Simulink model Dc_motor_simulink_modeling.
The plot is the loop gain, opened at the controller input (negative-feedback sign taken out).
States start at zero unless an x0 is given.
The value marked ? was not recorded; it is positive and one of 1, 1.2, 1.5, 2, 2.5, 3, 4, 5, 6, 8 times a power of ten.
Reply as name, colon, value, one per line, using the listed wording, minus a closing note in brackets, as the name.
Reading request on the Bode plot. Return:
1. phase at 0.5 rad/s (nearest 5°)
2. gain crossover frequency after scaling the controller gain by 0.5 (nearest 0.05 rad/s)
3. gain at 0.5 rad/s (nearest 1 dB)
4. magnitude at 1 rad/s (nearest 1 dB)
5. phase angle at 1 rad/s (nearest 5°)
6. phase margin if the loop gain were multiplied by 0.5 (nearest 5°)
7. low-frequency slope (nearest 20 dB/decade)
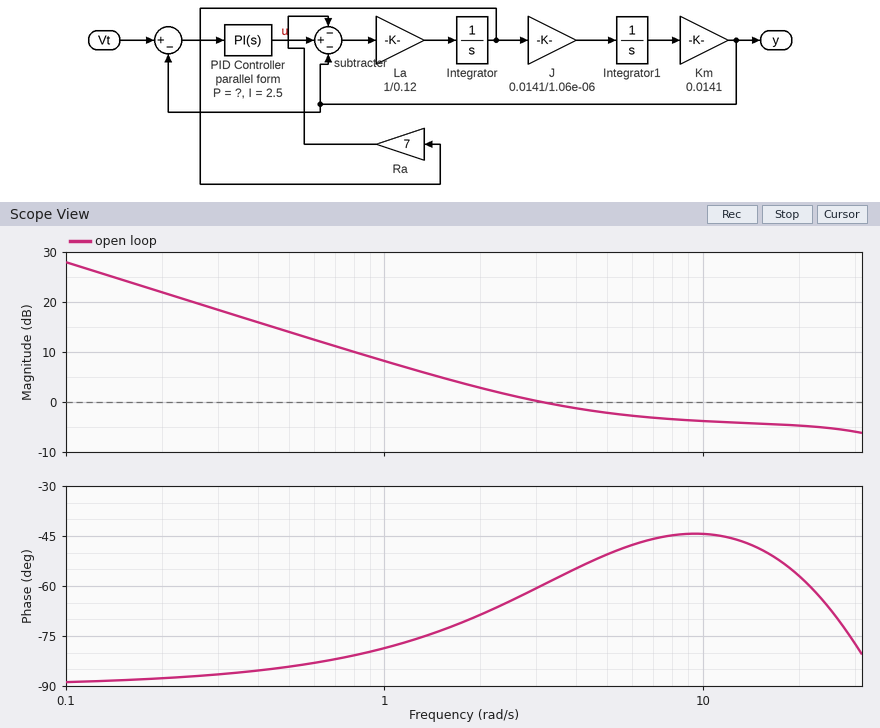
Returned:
phase at 0.5 rad/s: -85°
gain crossover frequency after scaling the controller gain by 0.5: 1.30 rad/s
gain at 0.5 rad/s: 14 dB
magnitude at 1 rad/s: 8 dB
phase angle at 1 rad/s: -80°
phase margin if the loop gain were multiplied by 0.5: 105°
low-frequency slope: -20 dB/decade
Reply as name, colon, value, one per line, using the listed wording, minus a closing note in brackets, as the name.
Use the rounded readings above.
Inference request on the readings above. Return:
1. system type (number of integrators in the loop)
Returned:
system type: 1
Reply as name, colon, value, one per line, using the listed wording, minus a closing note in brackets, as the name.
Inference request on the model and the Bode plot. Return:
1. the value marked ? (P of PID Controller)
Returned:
the value marked ?: 0.6
